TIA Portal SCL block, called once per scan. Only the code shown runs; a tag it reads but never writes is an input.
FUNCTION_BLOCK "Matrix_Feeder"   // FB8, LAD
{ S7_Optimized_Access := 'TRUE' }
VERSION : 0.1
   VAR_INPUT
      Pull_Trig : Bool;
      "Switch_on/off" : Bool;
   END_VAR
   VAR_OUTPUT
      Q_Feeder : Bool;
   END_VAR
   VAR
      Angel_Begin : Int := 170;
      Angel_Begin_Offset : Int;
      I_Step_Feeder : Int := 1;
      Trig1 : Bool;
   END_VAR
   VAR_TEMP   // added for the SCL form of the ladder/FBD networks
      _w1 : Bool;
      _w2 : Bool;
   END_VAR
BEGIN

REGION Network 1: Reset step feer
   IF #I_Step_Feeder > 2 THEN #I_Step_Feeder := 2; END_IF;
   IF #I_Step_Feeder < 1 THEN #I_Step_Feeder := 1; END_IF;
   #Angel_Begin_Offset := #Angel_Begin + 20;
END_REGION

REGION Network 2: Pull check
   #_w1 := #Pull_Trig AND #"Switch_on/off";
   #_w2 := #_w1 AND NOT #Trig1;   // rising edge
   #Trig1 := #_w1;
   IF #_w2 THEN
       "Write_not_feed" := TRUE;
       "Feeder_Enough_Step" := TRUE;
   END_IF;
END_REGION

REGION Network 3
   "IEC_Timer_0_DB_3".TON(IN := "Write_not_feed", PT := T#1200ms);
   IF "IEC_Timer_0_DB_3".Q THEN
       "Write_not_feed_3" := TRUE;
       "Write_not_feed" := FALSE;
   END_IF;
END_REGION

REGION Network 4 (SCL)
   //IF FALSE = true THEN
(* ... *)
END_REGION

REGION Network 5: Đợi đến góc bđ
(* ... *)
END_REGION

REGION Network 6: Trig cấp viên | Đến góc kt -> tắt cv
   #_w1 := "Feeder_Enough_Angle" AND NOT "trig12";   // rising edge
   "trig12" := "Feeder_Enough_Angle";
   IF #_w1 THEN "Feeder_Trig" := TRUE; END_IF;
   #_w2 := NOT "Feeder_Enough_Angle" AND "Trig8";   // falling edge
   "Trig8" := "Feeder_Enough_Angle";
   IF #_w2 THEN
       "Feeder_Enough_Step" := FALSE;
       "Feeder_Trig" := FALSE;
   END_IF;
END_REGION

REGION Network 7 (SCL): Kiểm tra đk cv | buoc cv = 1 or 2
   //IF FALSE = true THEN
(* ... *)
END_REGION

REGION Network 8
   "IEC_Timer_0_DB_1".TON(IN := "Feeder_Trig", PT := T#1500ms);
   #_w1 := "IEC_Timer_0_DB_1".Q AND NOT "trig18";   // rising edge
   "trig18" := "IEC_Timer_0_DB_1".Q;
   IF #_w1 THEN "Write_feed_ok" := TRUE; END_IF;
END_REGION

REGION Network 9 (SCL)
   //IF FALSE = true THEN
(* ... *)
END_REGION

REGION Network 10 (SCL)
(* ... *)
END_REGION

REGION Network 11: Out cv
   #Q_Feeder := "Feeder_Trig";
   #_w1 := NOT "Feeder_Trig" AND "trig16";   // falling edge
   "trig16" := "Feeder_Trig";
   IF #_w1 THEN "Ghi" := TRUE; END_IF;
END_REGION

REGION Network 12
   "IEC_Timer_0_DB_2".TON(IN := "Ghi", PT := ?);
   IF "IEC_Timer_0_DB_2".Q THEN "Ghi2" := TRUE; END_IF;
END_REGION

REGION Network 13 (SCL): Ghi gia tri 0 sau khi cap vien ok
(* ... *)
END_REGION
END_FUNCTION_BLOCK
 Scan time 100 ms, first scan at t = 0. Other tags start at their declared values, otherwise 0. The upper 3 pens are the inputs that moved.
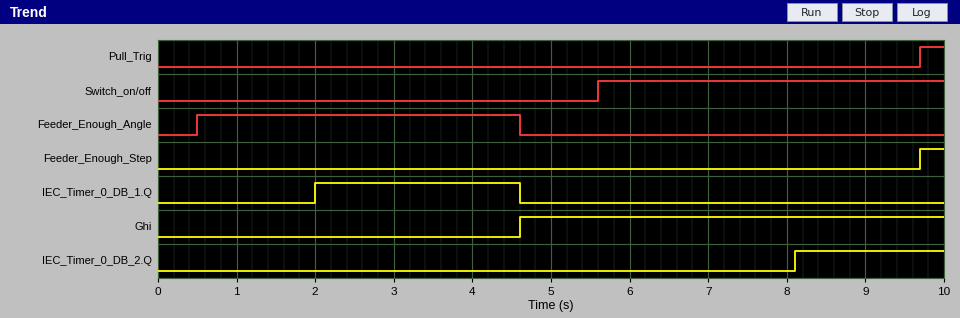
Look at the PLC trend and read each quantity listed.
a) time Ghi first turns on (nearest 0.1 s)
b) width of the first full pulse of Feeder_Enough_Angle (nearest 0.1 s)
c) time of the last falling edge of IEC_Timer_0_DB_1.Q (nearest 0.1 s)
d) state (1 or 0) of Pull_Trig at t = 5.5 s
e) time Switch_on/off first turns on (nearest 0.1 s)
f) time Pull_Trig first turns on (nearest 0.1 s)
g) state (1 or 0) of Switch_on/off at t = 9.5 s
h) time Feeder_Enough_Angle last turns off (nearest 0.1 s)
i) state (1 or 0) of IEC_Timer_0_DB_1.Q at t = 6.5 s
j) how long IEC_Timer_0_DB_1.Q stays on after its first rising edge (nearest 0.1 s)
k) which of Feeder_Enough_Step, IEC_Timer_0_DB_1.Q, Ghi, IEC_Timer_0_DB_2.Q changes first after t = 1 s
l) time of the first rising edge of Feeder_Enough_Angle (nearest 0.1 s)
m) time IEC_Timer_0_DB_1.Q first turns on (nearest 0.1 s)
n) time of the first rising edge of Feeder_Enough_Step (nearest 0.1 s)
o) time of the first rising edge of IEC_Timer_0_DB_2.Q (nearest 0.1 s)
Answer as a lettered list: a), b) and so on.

a) 4.6 s
b) 4.1 s
c) 4.6 s
d) 0
e) 5.6 s
f) 9.7 s
g) 1
h) 4.6 s
i) 0
j) 2.6 s
k) IEC_Timer_0_DB_1.Q
l) 0.5 s
m) 2.0 s
n) 9.7 s
o) 8.1 s
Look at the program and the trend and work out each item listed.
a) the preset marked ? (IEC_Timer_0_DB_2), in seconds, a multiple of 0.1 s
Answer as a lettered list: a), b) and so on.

a) 3.5 s
